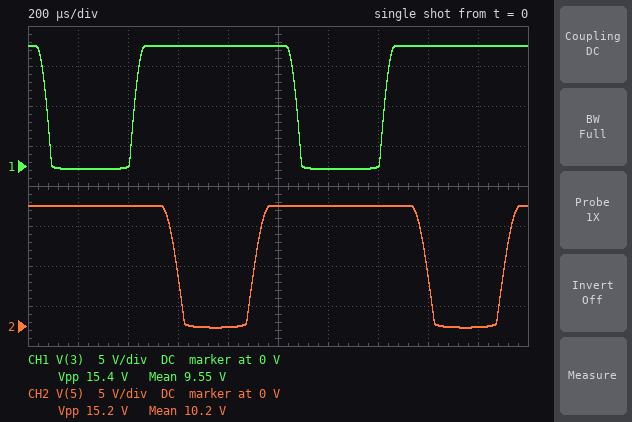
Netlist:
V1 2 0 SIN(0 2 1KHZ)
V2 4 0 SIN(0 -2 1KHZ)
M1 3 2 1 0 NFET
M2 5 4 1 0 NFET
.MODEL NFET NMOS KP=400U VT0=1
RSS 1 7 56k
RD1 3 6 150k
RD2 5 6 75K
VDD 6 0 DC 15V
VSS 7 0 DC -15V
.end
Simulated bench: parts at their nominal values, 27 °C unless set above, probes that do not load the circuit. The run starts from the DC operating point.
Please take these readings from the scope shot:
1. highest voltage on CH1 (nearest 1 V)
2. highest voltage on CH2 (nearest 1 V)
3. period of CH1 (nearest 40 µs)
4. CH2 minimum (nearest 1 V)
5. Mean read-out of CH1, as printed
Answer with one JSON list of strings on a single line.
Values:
["15 V", "15 V", "1.00 ms", "0 V", "9.55 V"]
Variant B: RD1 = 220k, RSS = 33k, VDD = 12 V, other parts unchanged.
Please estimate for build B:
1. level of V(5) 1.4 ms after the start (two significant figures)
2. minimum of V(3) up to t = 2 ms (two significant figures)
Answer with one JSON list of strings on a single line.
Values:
["12 V", "-510 mV"]
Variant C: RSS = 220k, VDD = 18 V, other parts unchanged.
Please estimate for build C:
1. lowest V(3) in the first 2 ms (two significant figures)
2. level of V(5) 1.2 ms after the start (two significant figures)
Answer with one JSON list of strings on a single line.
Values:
["7.5 V", "18 V"]
